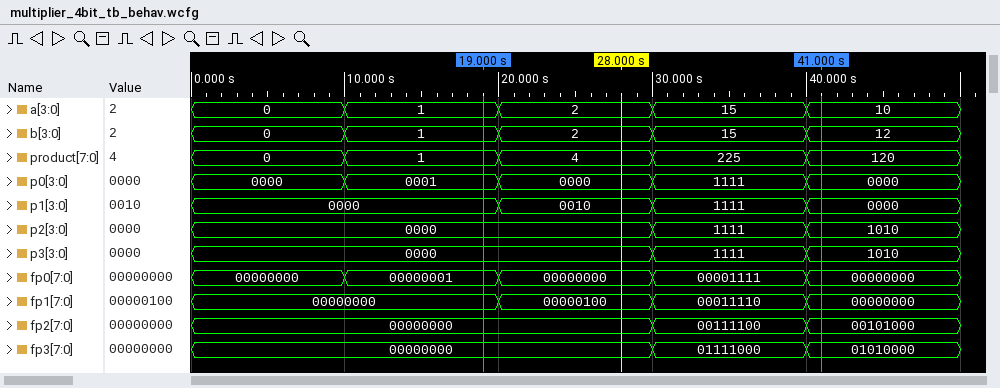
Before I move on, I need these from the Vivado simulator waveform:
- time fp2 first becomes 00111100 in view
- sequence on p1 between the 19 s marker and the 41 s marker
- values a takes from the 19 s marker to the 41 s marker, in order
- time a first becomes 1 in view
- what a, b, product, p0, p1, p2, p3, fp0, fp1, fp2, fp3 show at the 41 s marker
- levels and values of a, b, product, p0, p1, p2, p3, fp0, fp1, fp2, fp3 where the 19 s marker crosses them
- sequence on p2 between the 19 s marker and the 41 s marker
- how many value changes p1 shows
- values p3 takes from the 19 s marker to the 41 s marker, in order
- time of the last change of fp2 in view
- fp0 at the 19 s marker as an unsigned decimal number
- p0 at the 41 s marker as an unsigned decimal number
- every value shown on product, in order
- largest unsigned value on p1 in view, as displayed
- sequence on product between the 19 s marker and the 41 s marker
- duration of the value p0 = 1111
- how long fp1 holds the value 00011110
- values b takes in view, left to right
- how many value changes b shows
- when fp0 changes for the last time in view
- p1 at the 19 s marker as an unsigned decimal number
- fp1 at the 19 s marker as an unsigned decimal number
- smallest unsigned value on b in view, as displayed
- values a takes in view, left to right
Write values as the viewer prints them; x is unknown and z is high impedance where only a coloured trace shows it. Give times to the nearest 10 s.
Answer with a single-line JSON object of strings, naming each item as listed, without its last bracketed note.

{"time fp2 first becomes 00111100 in view": "30 s", "sequence on p1 between the 19 s marker and the 41 s marker": "0000, 0010, 1111, 0000", "values a takes from the 19 s marker to the 41 s marker, in order": "1, 2, 15, 10", "time a first becomes 1 in view": "10 s", "what a, b, product, p0, p1, p2, p3, fp0, fp1, fp2, fp3 show at the 41 s marker": "a=10, b=12, product=120, p0=0000, p1=0000, p2=1010, p3=1010, fp0=00000000, fp1=00000000, fp2=00101000, fp3=01010000", "levels and values of a, b, product, p0, p1, p2, p3, fp0, fp1, fp2, fp3 where the 19 s marker crosses them": "a=1, b=1, product=1, p0=0001, p1=0000, p2=0000, p3=0000, fp0=00000001, fp1=00000000, fp2=00000000, fp3=00000000", "sequence on p2 between the 19 s marker and the 41 s marker": "0000, 1111, 1010", "how many value changes p1 shows": "3", "values p3 takes from the 19 s marker to the 41 s marker, in order": "0000, 1111, 1010", "time of the last change of fp2 in view": "40 s", "fp0 at the 19 s marker as an unsigned decimal number": "1", "p0 at the 41 s marker as an unsigned decimal number": "0", "every value shown on product, in order": "0, 1, 4, 225, 120", "largest unsigned value on p1 in view, as displayed": "1111", "sequence on product between the 19 s marker and the 41 s marker": "1, 4, 225, 120", "duration of the value p0 = 1111": "10 s", "how long fp1 holds the value 00011110": "10 s", "values b takes in view, left to right": "0, 1, 2, 15, 12", "how many value changes b shows": "4", "when fp0 changes for the last time in view": "40 s", "p1 at the 19 s marker as an unsigned decimal number": "0", "fp1 at the 19 s marker as an unsigned decimal number": "0", "smallest unsigned value on b in view, as displayed": "0", "values a takes in view, left to right": "0, 1, 2, 15, 10"}
